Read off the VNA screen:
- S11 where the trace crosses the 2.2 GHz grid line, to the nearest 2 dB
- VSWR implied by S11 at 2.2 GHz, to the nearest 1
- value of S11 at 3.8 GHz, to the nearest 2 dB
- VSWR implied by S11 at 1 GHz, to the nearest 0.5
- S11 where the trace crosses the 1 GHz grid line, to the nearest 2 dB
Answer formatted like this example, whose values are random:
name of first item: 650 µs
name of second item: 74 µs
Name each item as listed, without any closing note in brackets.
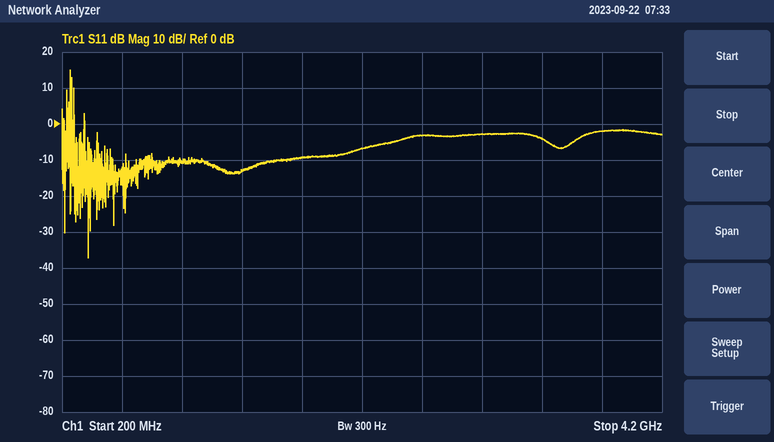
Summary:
S11 where the trace crosses the 2.2 GHz grid line, to the nearest 2 dB: -6 dB
VSWR implied by S11 at 2.2 GHz, to the nearest 1: 3
value of S11 at 3.8 GHz, to the nearest 2 dB: -2 dB
VSWR implied by S11 at 1 GHz, to the nearest 0.5: 2.0
S11 where the trace crosses the 1 GHz grid line, to the nearest 2 dB: -10 dB
